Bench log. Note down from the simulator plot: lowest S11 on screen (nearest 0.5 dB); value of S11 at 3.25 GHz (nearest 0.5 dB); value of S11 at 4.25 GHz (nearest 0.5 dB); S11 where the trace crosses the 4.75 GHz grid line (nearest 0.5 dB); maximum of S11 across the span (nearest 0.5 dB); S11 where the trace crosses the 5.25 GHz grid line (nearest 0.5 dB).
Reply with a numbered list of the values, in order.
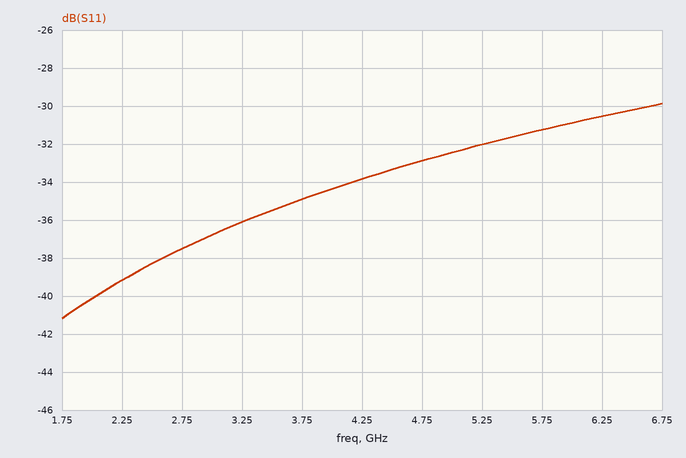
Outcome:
1. -41.0 dB
2. -36.0 dB
3. -34.0 dB
4. -33.0 dB
5. -30.0 dB
6. -32.0 dB
